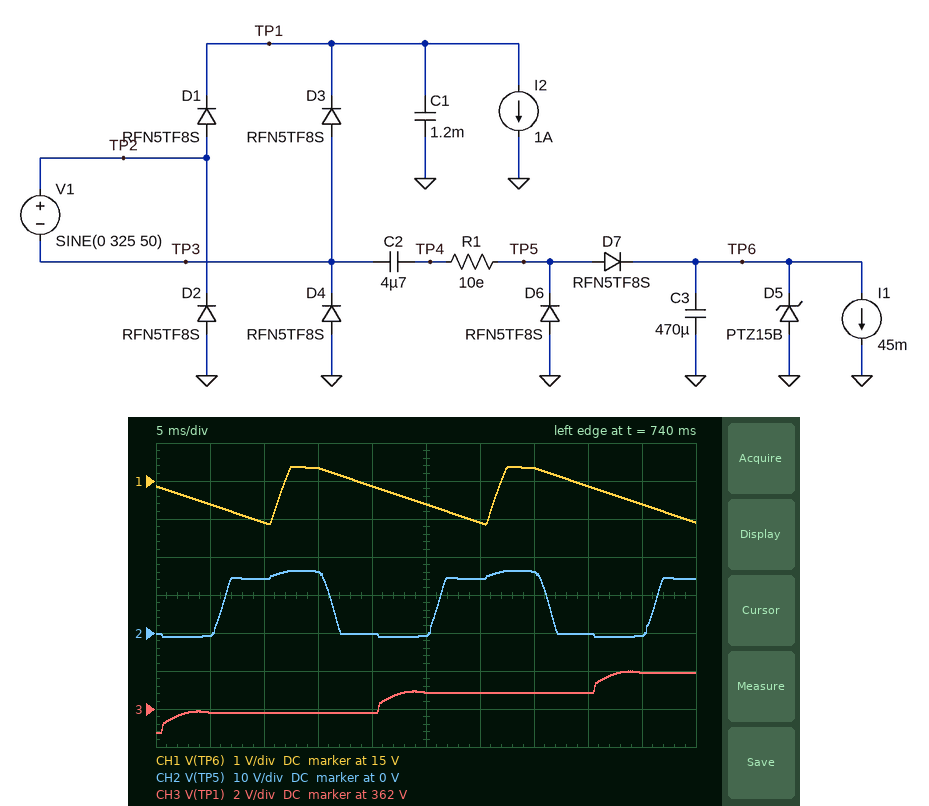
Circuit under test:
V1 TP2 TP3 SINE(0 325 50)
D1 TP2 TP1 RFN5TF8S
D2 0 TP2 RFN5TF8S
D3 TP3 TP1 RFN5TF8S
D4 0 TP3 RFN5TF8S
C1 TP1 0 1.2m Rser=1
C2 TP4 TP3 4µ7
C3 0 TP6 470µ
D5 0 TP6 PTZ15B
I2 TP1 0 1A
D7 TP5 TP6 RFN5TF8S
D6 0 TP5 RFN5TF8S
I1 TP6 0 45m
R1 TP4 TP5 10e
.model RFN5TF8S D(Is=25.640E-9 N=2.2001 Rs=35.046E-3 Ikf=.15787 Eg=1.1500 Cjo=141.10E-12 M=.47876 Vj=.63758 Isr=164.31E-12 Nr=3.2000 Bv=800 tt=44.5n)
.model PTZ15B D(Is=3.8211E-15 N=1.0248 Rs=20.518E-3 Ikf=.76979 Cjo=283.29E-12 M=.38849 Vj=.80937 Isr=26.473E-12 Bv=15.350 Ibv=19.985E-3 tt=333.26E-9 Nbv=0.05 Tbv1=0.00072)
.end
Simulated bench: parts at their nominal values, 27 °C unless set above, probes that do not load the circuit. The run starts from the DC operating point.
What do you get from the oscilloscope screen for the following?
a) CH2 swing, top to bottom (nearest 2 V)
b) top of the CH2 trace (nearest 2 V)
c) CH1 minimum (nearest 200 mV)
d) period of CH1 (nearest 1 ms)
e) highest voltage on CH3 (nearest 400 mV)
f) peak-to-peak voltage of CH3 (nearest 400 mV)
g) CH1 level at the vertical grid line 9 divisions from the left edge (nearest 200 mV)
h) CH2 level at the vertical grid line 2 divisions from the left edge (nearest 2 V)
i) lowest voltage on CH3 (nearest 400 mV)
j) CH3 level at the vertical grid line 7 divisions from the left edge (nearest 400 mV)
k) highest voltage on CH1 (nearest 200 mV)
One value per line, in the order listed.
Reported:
18 V
16 V
13.8 V
20 ms
364.0 V
3.2 V
14.4 V
14 V
360.8 V
362.8 V
15.4 V
